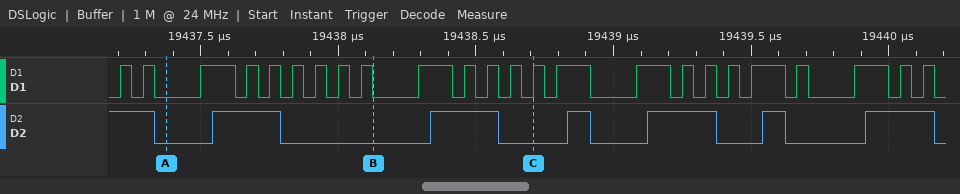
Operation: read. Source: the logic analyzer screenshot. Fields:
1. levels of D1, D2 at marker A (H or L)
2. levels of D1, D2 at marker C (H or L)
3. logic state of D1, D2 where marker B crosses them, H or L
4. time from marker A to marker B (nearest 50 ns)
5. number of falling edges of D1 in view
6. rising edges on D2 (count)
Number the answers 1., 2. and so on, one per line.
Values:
1. D1=L, D2=L
2. D1=H, D2=L
3. D1=L, D2=L
4. 750 ns
5. 24
6. 6
